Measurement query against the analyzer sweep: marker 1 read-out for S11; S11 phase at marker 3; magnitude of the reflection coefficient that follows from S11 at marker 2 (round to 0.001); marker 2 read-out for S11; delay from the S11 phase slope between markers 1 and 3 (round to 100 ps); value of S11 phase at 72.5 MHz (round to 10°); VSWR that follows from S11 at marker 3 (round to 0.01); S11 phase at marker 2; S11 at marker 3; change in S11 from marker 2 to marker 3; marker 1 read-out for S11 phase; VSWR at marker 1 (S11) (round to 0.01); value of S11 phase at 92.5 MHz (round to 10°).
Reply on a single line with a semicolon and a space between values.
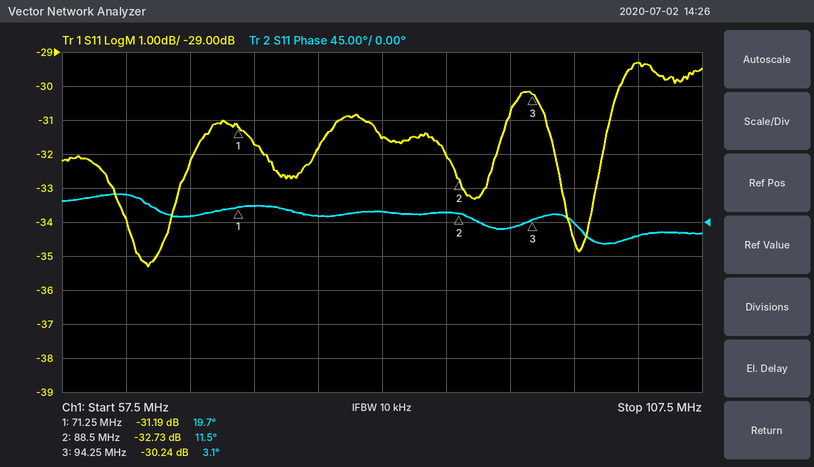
-31.19 dB; 3.1°; 0.023; -32.73 dB; 2.0 ns; 20°; 1.06; 11.5°; -30.24 dB; 2.49 dB; 19.7°; 1.06; -10°
